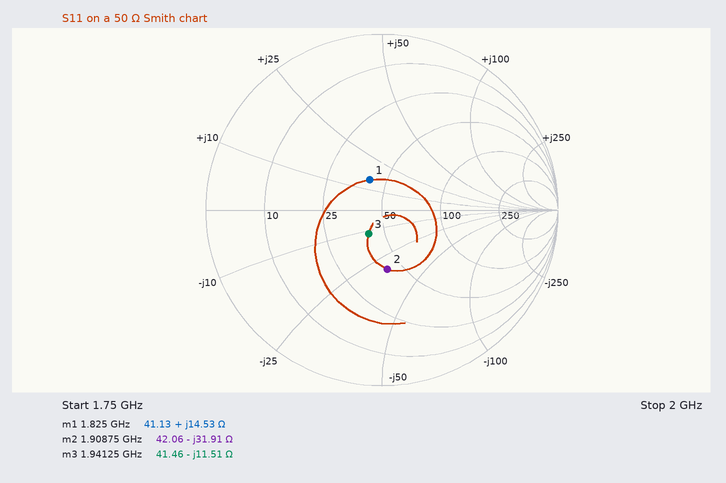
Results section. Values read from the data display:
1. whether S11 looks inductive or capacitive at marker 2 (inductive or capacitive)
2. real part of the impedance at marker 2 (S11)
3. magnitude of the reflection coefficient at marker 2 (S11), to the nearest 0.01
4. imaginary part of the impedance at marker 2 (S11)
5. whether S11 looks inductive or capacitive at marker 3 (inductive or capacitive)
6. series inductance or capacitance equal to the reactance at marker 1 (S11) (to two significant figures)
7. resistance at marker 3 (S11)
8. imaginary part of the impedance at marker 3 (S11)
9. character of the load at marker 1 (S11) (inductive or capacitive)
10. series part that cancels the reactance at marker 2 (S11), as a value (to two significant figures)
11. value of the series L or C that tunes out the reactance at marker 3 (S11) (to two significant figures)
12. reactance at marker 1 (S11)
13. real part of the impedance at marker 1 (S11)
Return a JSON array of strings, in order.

["capacitive", "42.06 Ω", "0.34", "-31.91 Ω", "capacitive", "1.3 nH", "41.46 Ω", "-11.51 Ω", "inductive", "2.7 nH", "940 pH", "+14.53 Ω", "41.13 Ω"]
